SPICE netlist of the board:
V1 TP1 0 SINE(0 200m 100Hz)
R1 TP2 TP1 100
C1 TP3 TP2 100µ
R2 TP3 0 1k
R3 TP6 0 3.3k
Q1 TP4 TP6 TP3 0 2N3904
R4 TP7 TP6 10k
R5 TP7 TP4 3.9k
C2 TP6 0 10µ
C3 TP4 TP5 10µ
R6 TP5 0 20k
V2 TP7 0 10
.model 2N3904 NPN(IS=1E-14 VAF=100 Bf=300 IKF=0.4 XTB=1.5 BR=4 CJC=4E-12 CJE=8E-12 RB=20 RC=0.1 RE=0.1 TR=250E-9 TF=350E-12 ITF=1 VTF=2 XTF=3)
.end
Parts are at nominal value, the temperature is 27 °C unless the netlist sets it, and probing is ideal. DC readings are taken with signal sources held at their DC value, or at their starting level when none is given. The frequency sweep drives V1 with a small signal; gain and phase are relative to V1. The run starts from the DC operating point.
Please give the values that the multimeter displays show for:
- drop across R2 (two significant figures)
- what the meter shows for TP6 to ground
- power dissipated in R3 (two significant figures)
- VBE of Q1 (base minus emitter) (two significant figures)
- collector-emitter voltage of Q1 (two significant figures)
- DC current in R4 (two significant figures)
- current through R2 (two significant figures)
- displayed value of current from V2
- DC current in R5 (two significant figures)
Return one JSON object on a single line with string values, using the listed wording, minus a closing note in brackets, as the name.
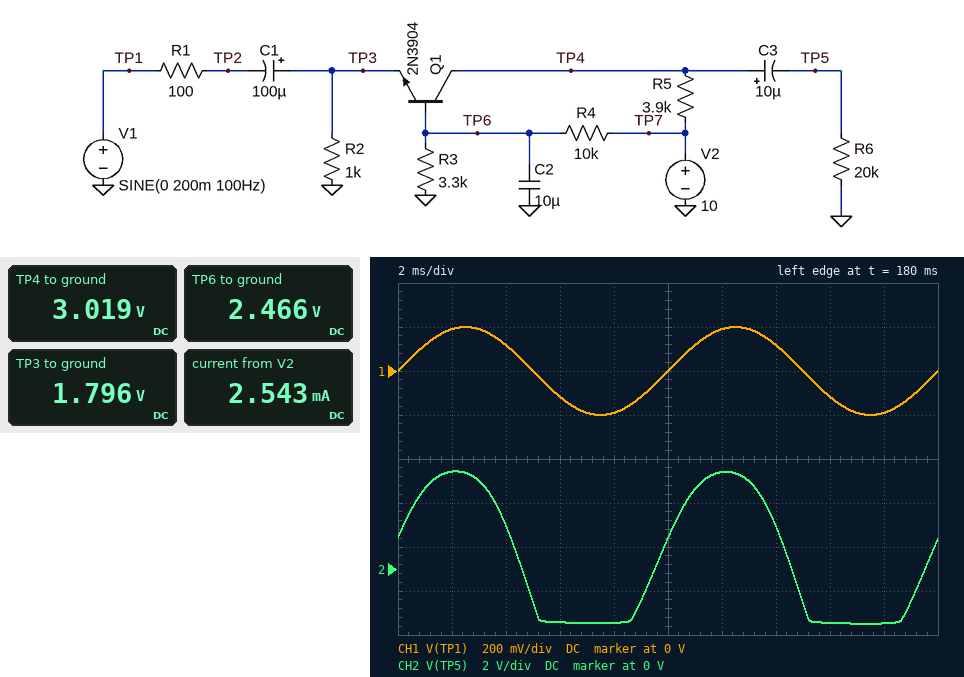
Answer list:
{"drop across R2": "1.8 V", "what the meter shows for TP6 to ground": "2.466 V", "power dissipated in R3": "1.8 mW", "VBE of Q1 (base minus emitter)": "670 mV", "collector-emitter voltage of Q1": "1.2 V", "DC current in R4": "750 µA", "current through R2": "1.8 mA", "displayed value of current from V2": "2.543 mA", "DC current in R5": "1.8 mA"}
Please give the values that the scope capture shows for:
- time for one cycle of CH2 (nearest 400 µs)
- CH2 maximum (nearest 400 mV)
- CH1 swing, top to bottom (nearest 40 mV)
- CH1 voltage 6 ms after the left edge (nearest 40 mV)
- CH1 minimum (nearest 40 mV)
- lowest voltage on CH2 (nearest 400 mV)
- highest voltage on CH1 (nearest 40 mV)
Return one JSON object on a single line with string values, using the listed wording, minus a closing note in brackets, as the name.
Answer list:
{"time for one cycle of CH2": "10.0 ms", "CH2 maximum": "4.4 V", "CH1 swing, top to bottom": "400 mV", "CH1 voltage 6 ms after the left edge": "-120 mV", "CH1 minimum": "-200 mV", "lowest voltage on CH2": "-2.4 V", "highest voltage on CH1": "200 mV"}
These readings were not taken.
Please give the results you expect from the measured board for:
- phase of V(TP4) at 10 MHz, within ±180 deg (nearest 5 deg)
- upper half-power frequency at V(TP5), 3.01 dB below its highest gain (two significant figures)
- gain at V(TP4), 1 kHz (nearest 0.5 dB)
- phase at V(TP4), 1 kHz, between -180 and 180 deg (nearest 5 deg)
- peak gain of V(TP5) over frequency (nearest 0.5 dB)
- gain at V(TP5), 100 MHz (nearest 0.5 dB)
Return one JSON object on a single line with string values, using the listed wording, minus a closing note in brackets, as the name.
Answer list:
{"phase of V(TP4) at 10 MHz, within ±180 deg": "-40 deg", "upper half-power frequency at V(TP5), 3.01 dB below its highest gain": "12 MHz", "gain at V(TP4), 1 kHz": "29.0 dB", "phase at V(TP4), 1 kHz, between -180 and 180 deg": "0 deg", "peak gain of V(TP5) over frequency": "29.0 dB", "gain at V(TP5), 100 MHz": "10.0 dB"}
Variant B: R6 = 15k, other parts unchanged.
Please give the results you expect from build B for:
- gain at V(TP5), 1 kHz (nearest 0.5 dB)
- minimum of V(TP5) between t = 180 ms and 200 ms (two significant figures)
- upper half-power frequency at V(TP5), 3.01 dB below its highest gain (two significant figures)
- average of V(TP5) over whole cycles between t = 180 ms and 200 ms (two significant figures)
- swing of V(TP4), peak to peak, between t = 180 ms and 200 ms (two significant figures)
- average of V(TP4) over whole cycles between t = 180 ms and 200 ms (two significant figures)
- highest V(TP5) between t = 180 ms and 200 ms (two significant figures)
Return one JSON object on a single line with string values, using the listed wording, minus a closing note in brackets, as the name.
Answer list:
{"gain at V(TP5), 1 kHz": "28.5 dB", "minimum of V(TP5) between t = 180 ms and 200 ms": "-2.6 V", "upper half-power frequency at V(TP5), 3.01 dB below its highest gain": "13 MHz", "average of V(TP5) over whole cycles between t = 180 ms and 200 ms": "350 mV", "swing of V(TP4), peak to peak, between t = 180 ms and 200 ms": "6.7 V", "average of V(TP4) over whole cycles between t = 180 ms and 200 ms": "4.4 V", "highest V(TP5) between t = 180 ms and 200 ms": "4.1 V"}
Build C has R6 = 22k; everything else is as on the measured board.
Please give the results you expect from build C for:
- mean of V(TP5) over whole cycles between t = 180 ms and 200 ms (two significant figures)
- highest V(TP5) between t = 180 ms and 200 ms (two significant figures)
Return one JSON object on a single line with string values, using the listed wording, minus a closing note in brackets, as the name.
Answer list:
{"mean of V(TP5) over whole cycles between t = 180 ms and 200 ms": "570 mV", "highest V(TP5) between t = 180 ms and 200 ms": "4.5 V"}
